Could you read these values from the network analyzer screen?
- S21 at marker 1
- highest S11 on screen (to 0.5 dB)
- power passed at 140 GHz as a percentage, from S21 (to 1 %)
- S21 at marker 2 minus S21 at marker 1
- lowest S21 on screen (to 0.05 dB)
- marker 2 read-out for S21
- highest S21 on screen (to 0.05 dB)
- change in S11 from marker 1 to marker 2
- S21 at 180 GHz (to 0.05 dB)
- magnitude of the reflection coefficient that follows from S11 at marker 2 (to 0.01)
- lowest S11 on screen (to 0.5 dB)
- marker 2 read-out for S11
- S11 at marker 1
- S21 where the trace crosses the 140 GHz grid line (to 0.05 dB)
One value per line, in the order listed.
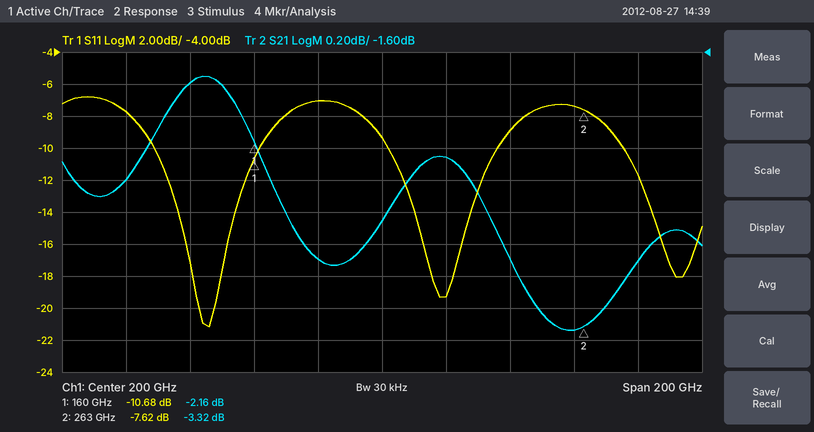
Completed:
-2.16 dB
-7.0 dB
66 %
-1.16 dB
-3.35 dB
-3.32 dB
-1.75 dB
3.06 dB
-2.90 dB
0.42
-21.0 dB
-7.62 dB
-10.68 dB
-1.80 dB
